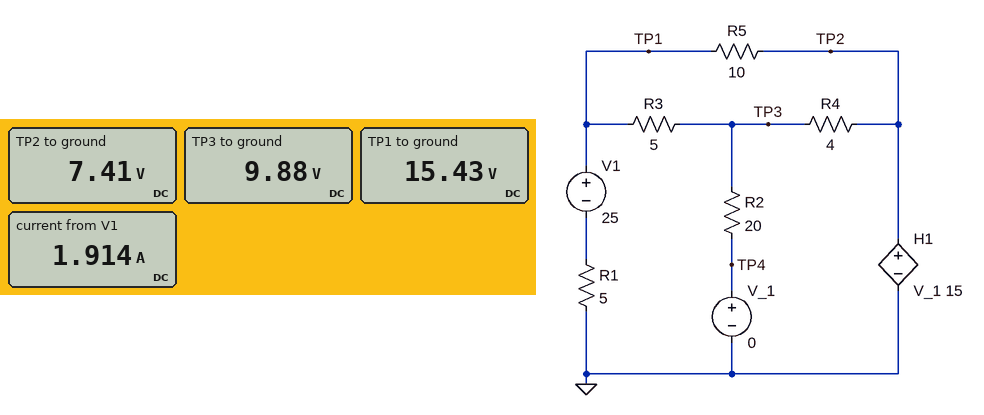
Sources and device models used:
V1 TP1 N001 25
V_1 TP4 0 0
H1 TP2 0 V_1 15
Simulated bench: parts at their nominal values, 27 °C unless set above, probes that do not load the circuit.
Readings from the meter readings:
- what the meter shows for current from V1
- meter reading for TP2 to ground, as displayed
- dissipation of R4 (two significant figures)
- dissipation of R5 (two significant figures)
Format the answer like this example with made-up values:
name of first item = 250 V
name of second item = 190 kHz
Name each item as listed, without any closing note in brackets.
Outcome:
what the meter shows for current from V1 = 1.914 A
meter reading for TP2 to ground, as displayed = 7.41 V
dissipation of R4 = 1.5 W
dissipation of R5 = 6.4 W
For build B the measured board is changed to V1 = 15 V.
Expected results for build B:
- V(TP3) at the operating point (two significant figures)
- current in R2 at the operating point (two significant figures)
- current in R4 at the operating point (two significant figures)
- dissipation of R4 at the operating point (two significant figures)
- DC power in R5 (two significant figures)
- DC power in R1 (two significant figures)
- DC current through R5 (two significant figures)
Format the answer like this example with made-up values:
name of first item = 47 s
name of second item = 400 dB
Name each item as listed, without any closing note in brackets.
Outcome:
V(TP3) at the operating point = 5.9 V
current in R2 at the operating point = 300 mA
current in R4 at the operating point = 370 mA
dissipation of R4 at the operating point = 550 mW
DC power in R5 = 2.3 W
DC power in R1 = 6.6 W
DC current through R5 = 480 mA
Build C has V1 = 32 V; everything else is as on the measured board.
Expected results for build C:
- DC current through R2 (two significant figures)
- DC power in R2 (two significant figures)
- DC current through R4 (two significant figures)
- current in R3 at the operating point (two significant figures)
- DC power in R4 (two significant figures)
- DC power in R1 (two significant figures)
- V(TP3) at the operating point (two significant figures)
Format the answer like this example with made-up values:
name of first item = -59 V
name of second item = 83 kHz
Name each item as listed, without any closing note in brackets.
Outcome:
DC current through R2 = 630 mA
DC power in R2 = 8.0 W
DC current through R4 = 790 mA
current in R3 at the operating point = 1.4 A
DC power in R4 = 2.5 W
DC power in R1 = 30 W
V(TP3) at the operating point = 13 V
